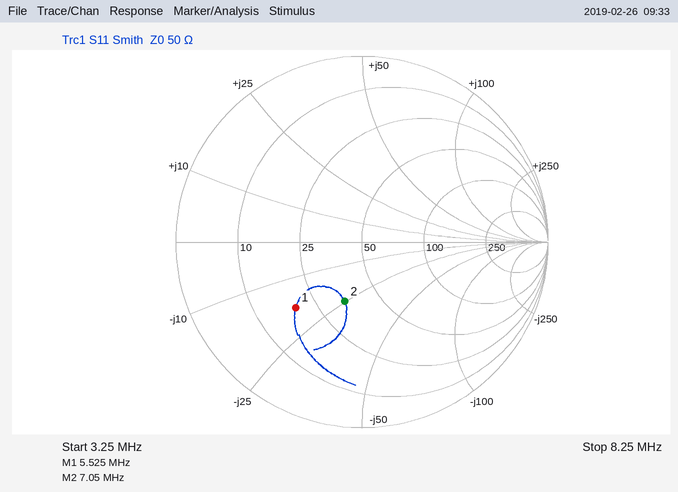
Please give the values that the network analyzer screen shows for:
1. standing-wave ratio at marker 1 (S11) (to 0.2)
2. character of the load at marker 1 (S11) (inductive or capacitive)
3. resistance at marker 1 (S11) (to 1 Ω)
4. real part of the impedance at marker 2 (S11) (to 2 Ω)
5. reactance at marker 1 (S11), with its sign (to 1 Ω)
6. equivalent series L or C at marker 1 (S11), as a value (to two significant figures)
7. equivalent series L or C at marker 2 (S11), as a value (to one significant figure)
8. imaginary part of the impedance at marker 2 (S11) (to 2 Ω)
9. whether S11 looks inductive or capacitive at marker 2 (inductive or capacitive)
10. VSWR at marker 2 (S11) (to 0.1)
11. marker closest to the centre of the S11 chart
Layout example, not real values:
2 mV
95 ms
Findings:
3.0
capacitive
19 Ω
34 Ω
-18 Ω
1.6 nF
900 pF
-24 Ω
capacitive
2.0
marker 2
